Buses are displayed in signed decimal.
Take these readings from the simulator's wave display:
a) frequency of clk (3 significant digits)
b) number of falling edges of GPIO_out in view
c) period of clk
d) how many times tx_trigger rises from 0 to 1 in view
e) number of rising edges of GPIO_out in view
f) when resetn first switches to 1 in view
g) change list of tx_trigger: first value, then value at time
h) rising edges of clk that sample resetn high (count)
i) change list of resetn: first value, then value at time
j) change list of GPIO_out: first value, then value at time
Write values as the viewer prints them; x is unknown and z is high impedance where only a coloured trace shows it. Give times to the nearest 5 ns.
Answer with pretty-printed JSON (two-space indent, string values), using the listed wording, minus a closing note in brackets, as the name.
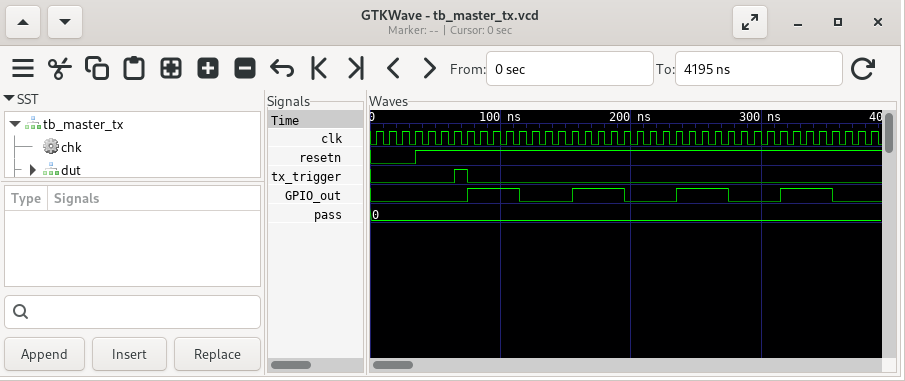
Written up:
{
  "frequency of clk": "100 MHz",
  "number of falling edges of GPIO_out in view": "4",
  "period of clk": "10 ns",
  "how many times tx_trigger rises from 0 to 1 in view": "1",
  "number of rising edges of GPIO_out in view": "4",
  "when resetn first switches to 1 in view": "35 ns",
  "change list of tx_trigger: first value, then value at time": "0, 1 at 65 ns, 0 at 75 ns",
  "rising edges of clk that sample resetn high": "35",
  "change list of resetn: first value, then value at time": "0, 1 at 35 ns",
  "change list of GPIO_out: first value, then value at time": "0, 1 at 75 ns, 0 at 115 ns, 1 at 155 ns, 0 at 195 ns, 1 at 235 ns, 0 at 275 ns, 1 at 315 ns, 0 at 355 ns"
}
